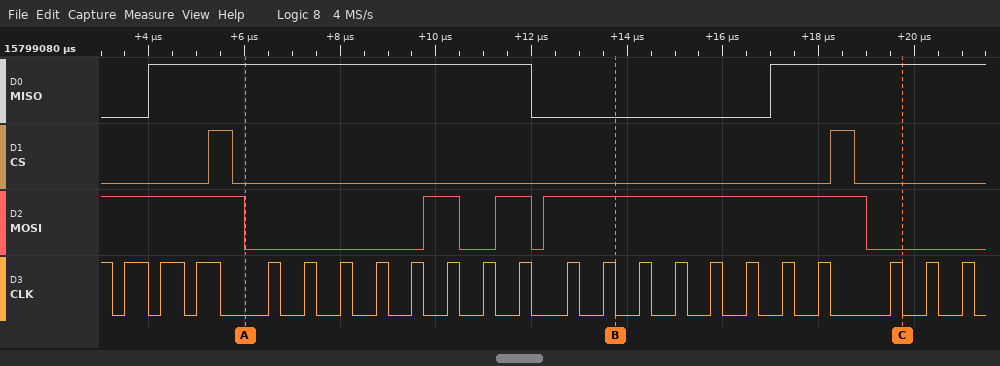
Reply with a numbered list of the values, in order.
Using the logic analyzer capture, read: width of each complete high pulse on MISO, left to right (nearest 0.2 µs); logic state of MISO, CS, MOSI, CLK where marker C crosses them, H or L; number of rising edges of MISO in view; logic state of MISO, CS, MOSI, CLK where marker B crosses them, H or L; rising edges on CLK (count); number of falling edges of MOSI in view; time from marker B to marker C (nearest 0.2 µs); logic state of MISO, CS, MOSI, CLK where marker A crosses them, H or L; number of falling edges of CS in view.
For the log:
1. 8 µs
2. MISO=H, CS=L, MOSI=L, CLK=L
3. 2
4. MISO=L, CS=L, MOSI=H, CLK=L
5. 22
6. 4
7. 6 µs
8. MISO=H, CS=L, MOSI=L, CLK=L
9. 2
